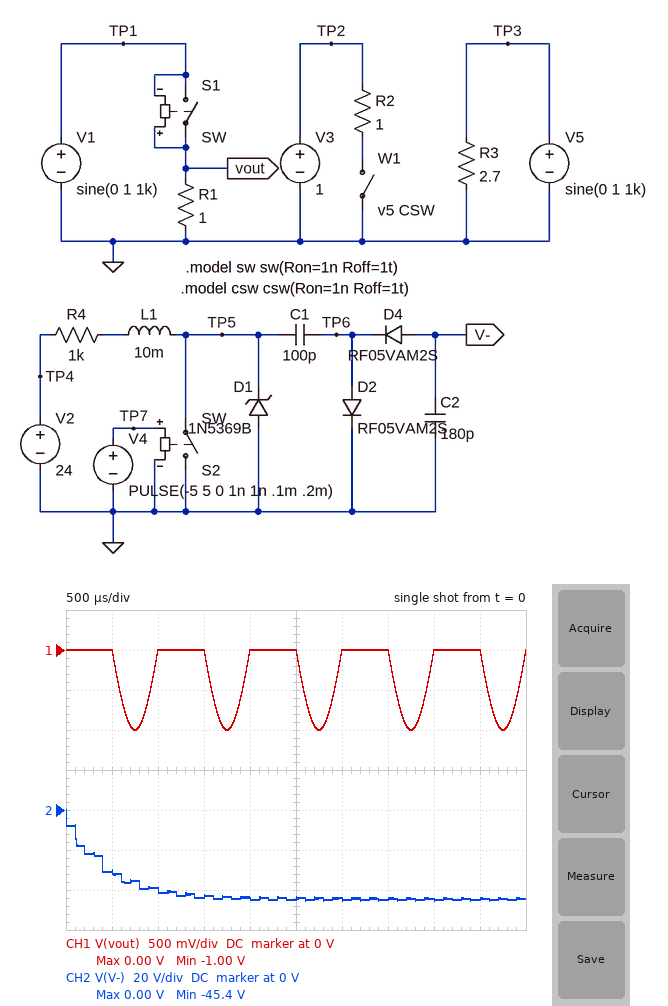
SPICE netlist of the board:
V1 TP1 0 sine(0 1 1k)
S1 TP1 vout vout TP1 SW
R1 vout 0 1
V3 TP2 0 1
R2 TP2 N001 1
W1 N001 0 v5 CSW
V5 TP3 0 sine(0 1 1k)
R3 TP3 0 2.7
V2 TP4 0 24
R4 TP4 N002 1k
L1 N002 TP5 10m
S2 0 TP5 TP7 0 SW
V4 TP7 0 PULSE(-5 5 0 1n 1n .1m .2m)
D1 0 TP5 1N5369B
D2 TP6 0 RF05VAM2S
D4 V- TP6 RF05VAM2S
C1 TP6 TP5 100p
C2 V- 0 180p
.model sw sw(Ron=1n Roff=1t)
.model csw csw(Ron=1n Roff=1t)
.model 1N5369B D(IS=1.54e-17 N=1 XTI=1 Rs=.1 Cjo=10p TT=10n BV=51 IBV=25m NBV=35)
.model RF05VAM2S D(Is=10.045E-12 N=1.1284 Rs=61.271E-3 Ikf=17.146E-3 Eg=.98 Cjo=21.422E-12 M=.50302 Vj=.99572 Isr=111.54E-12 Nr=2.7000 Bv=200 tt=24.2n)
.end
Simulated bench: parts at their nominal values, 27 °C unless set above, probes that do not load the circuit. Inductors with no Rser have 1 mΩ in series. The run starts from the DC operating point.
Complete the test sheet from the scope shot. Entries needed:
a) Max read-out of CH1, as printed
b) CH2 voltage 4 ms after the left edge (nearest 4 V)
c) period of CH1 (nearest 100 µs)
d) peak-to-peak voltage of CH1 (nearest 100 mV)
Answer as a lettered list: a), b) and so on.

a) 0.00 V
b) -44 V
c) 1.0 ms
d) 1.0 V
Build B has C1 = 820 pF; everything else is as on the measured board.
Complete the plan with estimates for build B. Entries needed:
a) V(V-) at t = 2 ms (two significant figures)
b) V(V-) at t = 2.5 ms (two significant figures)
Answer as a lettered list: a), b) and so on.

a) -49 V
b) -50 V
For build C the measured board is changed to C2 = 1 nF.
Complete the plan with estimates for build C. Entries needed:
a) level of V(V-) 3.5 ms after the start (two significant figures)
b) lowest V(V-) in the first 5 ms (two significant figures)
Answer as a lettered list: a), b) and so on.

a) -38 V
b) -42 V
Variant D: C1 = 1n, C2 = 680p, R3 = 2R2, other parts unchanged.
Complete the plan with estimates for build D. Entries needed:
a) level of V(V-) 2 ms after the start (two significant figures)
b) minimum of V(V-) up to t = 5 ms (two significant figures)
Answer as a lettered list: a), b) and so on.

a) -49 V
b) -50 V
